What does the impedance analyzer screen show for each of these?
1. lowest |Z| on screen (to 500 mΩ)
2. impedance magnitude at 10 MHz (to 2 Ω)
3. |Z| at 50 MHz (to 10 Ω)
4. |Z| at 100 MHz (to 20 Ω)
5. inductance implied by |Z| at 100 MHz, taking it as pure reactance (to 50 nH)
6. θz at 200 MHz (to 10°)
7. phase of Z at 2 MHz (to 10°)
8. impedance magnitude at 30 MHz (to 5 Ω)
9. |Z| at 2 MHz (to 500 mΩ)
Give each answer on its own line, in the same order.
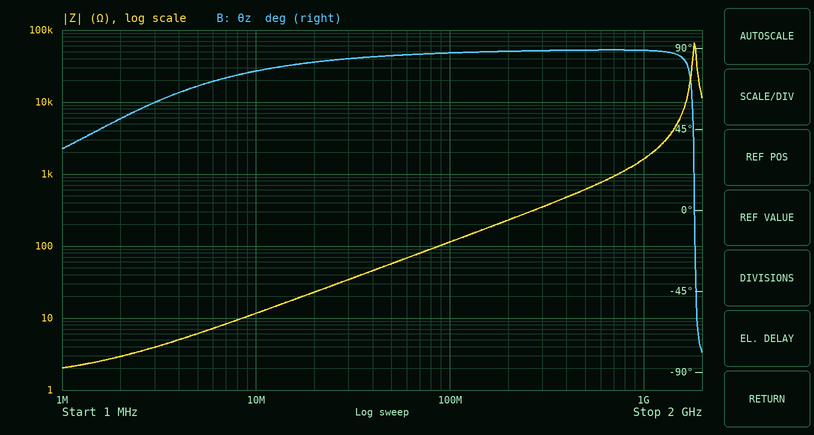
2.0 Ω
12 Ω
60 Ω
120 Ω
200 nH
90°
50°
35 Ω
3.0 Ω
